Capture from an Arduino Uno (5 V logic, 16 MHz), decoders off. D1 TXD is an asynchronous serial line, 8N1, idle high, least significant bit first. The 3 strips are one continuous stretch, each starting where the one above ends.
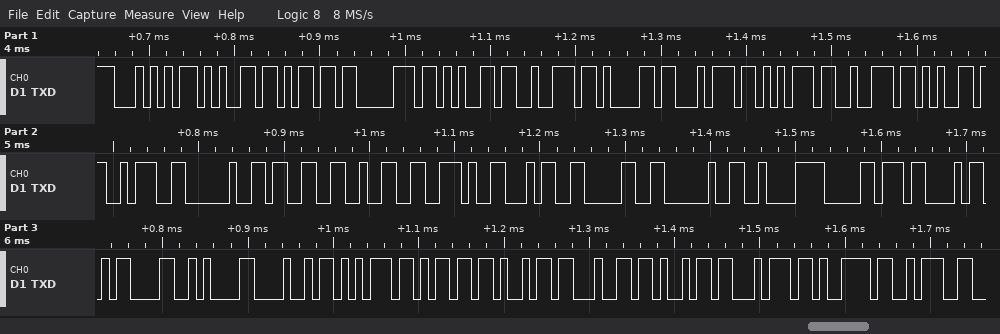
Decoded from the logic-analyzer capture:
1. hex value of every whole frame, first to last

0x54 0x65 0x6D 0x70 0x65 0x72 0x61 0x74 0x75 0x72 0x65 0x3A 0x20 0x33 0x32 0x2E 0x34 0x30 0x20 0xC2 0xB0 0x43 0x0D 0x0A 0x48 0x75 0x6D 0x69 0x64 0x69 0x74 0x79 0x3A
